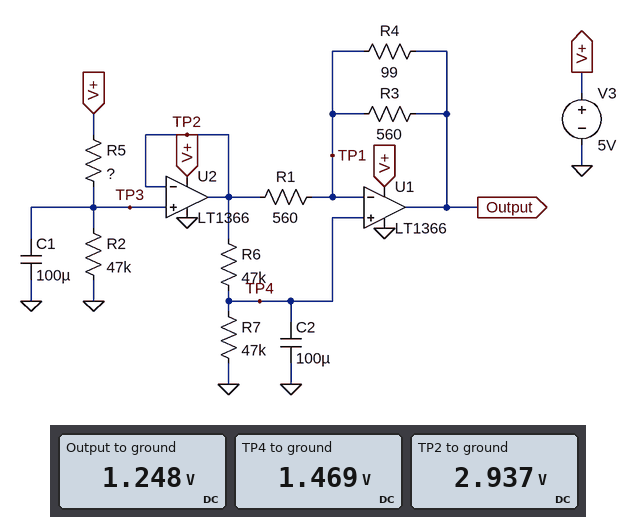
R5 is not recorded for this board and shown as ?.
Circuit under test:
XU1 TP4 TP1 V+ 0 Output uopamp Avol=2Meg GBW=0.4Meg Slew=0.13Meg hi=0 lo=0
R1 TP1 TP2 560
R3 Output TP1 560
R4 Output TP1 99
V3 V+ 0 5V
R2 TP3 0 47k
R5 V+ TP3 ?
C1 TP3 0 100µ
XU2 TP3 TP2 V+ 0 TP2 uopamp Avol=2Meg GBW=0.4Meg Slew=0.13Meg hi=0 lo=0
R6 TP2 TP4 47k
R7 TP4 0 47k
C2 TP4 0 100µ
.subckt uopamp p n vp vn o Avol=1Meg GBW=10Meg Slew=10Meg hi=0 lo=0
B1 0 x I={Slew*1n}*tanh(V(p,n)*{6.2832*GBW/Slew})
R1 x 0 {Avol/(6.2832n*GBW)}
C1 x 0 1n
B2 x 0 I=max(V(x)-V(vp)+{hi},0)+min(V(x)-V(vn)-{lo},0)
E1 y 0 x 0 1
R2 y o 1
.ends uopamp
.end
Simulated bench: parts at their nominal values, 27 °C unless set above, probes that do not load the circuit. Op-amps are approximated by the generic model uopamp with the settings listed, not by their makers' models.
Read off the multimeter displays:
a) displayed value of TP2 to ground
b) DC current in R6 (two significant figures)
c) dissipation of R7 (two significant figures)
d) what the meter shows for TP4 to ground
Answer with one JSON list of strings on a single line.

["2.937 V", "31 µA", "46 µW", "1.469 V"]
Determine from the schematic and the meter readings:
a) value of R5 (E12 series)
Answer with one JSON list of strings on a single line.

["33 kΩ"]
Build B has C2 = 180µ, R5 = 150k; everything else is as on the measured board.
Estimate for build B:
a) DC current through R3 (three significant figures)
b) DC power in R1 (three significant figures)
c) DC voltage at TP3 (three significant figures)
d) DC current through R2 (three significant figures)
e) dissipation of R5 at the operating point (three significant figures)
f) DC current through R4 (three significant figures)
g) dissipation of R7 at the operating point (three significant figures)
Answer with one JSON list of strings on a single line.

["160 µA", "635 µW", "1.19 V", "25.4 µA", "96.6 µW", "905 µA", "7.57 µW"]
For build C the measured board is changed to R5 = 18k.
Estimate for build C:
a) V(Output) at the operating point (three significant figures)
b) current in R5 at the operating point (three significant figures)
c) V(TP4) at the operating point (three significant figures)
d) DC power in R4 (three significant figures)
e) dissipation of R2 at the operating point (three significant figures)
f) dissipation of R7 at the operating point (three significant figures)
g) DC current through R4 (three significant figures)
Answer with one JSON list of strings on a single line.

["1.54 V", "76.9 µA", "1.81 V", "745 µW", "278 µW", "69.5 µW", "2.74 mA"]
